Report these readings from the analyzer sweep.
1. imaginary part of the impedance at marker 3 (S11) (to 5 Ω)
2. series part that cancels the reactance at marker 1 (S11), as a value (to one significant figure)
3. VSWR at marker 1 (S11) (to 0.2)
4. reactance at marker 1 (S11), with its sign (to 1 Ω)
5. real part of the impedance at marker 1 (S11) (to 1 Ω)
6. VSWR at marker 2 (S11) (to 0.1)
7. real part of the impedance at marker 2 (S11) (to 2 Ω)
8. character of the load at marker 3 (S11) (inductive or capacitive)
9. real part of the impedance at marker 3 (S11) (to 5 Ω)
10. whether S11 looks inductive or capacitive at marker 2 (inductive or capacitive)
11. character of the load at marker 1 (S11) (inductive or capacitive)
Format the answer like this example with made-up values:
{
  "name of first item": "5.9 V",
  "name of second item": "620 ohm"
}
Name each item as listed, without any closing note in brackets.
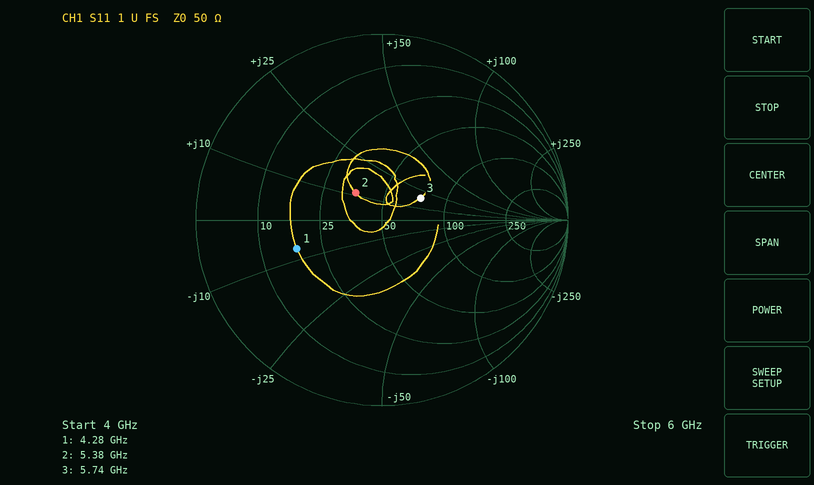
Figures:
{
  "imaginary part of the impedance at marker 3 (S11)": "+20 Ω",
  "series part that cancels the reactance at marker 1 (S11), as a value": "300 pH",
  "VSWR at marker 1 (S11)": "2.8",
  "reactance at marker 1 (S11), with its sign": "-7 Ω",
  "real part of the impedance at marker 1 (S11)": "18 Ω",
  "VSWR at marker 2 (S11)": "1.5",
  "real part of the impedance at marker 2 (S11)": "36 Ω",
  "character of the load at marker 3 (S11)": "inductive",
  "real part of the impedance at marker 3 (S11)": "75 Ω",
  "whether S11 looks inductive or capacitive at marker 2": "inductive",
  "character of the load at marker 1 (S11)": "capacitive"
}
